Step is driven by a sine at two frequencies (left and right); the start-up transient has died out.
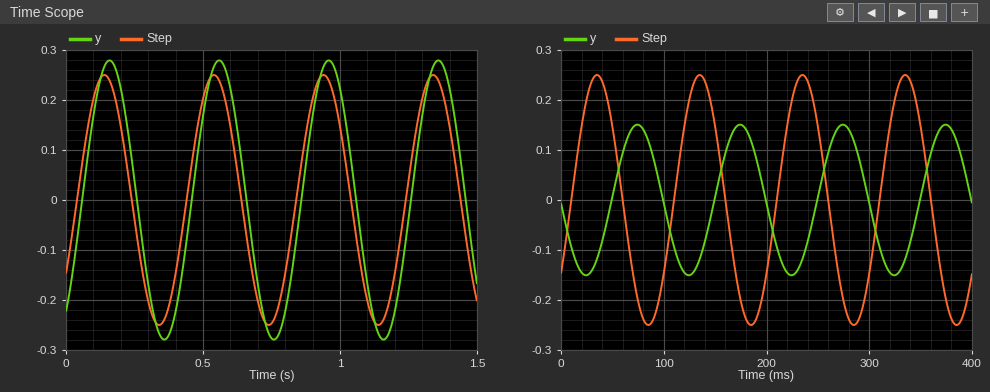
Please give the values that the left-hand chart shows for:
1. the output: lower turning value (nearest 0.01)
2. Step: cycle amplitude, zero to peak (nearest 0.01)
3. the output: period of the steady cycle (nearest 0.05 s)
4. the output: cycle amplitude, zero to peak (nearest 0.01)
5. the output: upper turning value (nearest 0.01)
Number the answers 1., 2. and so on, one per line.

1. -0.28
2. 0.25
3. 0.40 s
4. 0.28
5. 0.28
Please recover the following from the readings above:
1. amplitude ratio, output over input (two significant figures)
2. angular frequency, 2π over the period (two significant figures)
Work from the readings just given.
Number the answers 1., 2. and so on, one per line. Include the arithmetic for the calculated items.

1. 0.28 / 0.25 = 1.1
2. 2π / 0.4 = 16 rad/s
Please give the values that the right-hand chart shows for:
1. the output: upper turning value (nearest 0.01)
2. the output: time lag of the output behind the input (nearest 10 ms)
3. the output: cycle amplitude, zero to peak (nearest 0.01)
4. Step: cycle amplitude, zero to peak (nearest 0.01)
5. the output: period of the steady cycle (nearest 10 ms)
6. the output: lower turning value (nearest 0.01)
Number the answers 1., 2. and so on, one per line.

1. 0.15
2. 40 ms
3. 0.15
4. 0.25
5. 100 ms
6. -0.15
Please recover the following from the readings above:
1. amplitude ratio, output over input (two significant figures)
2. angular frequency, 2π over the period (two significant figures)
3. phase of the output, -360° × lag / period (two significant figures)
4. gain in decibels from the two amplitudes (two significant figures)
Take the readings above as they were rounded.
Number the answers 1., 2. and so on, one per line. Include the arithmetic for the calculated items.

1. 0.15 / 0.25 = 0.60
2. 2π / 100 = 0.063 rad/ms
3. -360 × 40 / 100 = -140°
4. 20 log10(0.15 / 0.25) = -4.4 dB
